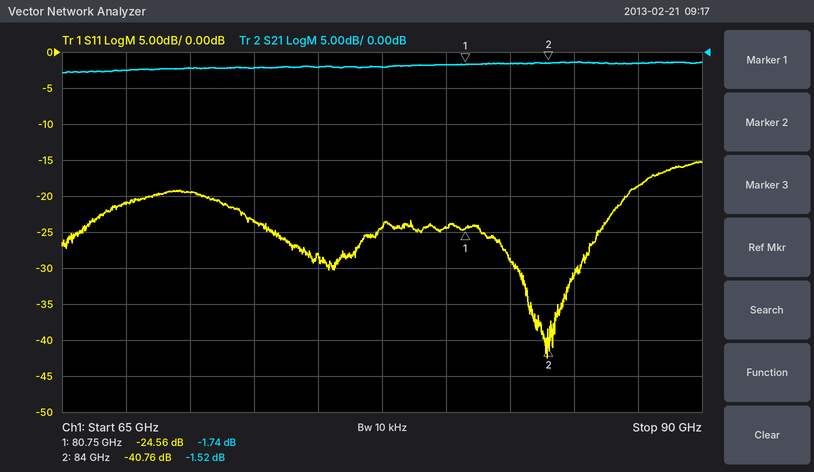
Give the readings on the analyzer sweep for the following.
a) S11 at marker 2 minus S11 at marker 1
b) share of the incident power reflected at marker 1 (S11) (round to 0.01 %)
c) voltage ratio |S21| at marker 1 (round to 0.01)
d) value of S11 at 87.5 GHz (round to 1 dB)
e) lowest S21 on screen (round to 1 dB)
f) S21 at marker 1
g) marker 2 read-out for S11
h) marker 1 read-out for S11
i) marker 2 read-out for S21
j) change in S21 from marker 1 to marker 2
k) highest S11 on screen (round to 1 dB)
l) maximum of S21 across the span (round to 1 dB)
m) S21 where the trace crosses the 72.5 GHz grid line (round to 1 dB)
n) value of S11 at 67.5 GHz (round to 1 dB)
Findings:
-16.20 dB
0.35 %
0.82
-19 dB
-3 dB
-1.74 dB
-40.76 dB
-24.56 dB
-1.52 dB
0.22 dB
-15 dB
-1 dB
-2 dB
-21 dB
